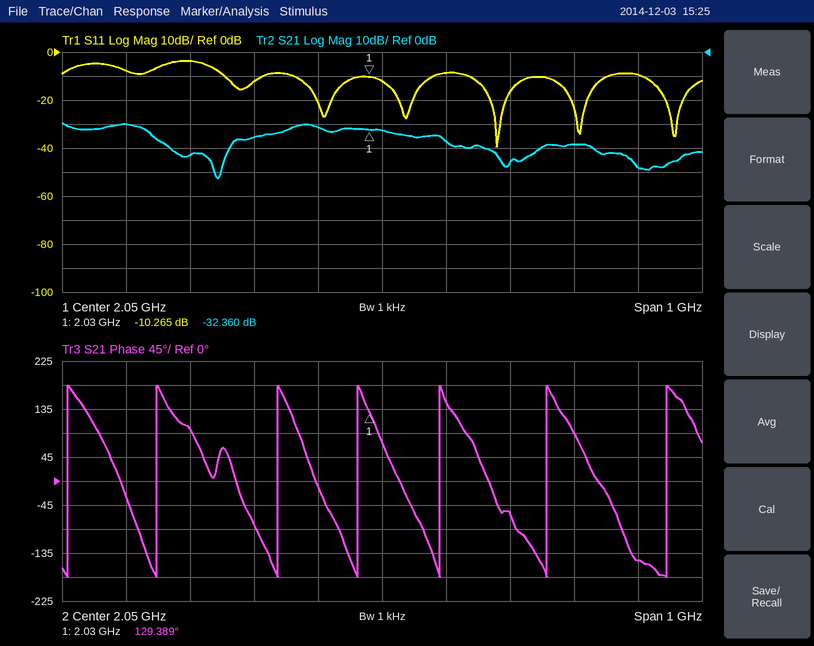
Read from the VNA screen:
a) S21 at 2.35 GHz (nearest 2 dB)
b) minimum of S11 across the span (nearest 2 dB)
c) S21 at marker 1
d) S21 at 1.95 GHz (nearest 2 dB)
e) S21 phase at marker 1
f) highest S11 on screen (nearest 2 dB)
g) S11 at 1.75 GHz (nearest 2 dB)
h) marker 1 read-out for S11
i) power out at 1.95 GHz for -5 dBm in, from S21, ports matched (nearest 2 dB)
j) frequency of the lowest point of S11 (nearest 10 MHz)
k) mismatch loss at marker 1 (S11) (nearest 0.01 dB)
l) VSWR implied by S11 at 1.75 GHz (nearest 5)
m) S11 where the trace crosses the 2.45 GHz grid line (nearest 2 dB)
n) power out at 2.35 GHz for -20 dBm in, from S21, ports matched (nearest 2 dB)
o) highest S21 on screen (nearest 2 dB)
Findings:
-38 dB
-40 dB
-32.360 dB
-32 dB
129.389°
-4 dB
-4 dB
-10.265 dB
-36 dBm
2.23 GHz
0.43 dB
5
-10 dB
-58 dBm
-30 dB
